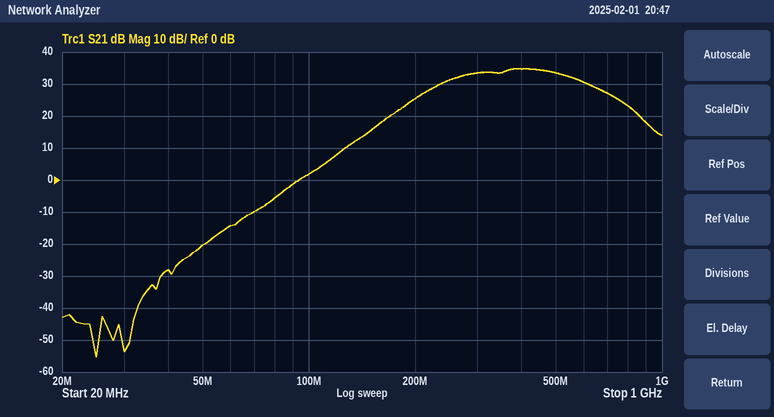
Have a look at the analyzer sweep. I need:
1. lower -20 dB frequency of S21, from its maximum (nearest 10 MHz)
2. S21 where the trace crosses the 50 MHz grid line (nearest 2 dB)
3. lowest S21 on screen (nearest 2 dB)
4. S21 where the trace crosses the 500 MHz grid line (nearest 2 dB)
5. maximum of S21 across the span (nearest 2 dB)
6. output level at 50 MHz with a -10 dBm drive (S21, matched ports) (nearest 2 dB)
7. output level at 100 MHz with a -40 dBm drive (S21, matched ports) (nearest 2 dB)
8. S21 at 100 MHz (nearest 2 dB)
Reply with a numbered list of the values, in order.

1. 150 MHz
2. -20 dB
3. -56 dB
4. 34 dB
5. 34 dB
6. -30 dBm
7. -38 dBm
8. 2 dB
